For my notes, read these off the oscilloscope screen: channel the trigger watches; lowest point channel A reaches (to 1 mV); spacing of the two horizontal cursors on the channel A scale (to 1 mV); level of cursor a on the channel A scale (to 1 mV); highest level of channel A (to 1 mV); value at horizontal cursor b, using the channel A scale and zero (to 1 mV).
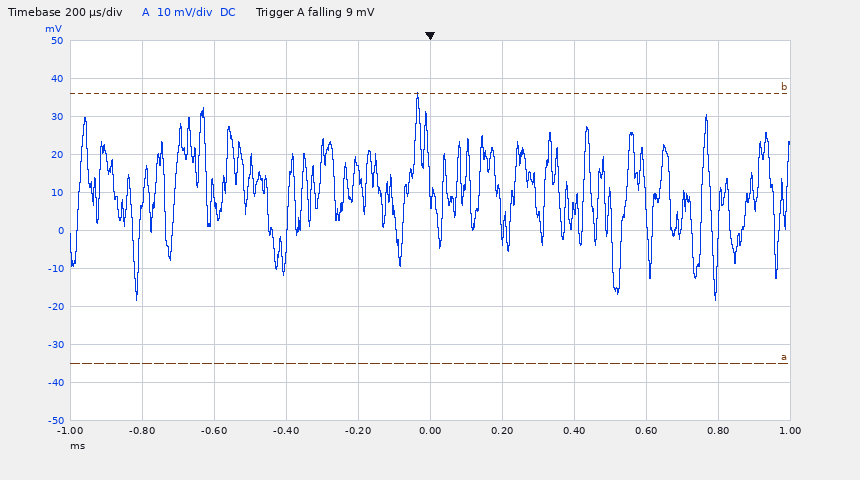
channel A
-18 mV
71 mV
-35 mV
36 mV
36 mV
